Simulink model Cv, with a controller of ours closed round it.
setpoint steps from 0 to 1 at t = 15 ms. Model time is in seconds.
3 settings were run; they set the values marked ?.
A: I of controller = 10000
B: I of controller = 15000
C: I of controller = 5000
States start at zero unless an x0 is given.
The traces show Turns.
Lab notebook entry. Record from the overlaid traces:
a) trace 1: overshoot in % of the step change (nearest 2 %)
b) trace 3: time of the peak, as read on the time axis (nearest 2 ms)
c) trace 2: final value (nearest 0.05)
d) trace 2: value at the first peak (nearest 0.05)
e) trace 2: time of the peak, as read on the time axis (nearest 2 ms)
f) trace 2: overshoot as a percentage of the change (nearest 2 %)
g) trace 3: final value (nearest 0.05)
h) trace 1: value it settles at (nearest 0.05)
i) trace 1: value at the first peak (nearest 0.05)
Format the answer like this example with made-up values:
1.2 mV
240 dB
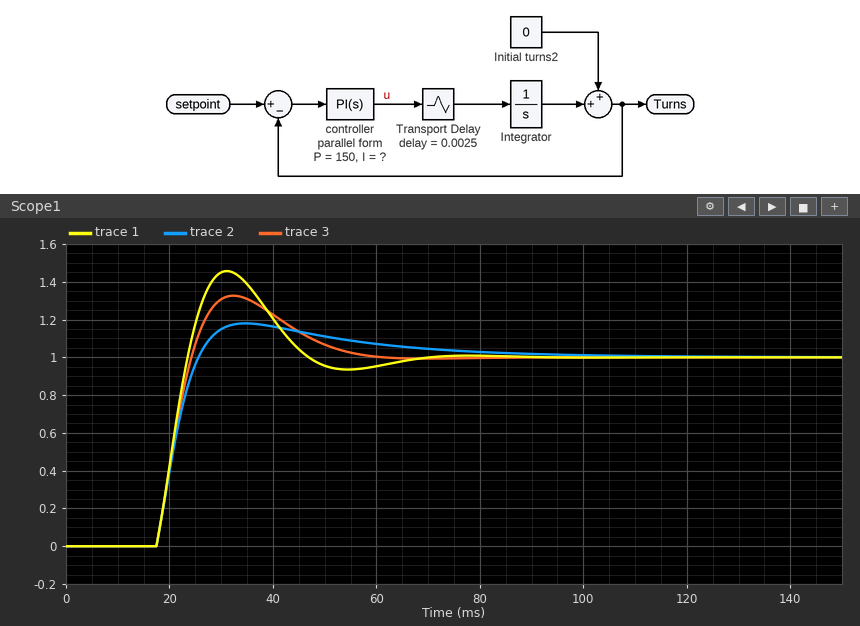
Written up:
46 %
32 ms
1.00
1.20
34 ms
18 %
1.00
1.00
1.45
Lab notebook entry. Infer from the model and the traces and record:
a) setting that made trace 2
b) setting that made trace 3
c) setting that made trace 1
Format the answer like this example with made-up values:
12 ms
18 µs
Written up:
C
A
B
